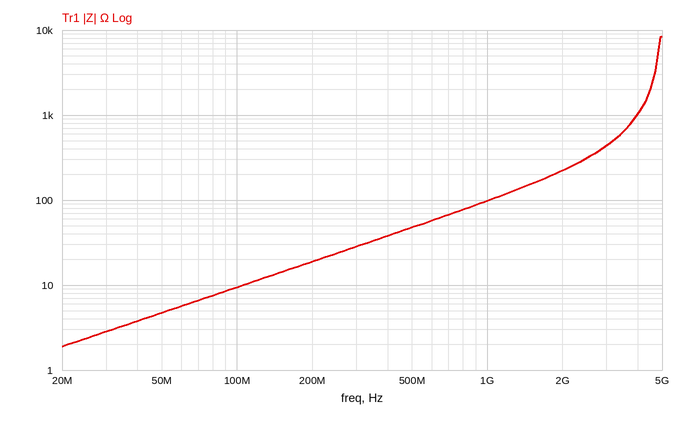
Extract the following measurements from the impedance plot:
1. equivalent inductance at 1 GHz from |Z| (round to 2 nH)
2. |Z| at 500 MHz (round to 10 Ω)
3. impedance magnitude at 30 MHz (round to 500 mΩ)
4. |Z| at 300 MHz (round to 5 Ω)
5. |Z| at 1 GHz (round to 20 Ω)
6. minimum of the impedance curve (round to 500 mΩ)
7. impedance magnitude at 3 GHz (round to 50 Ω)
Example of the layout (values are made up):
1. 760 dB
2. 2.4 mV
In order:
1. 16 nH
2. 50 Ω
3. 3.0 Ω
4. 30 Ω
5. 100 Ω
6. 2.0 Ω
7. 450 Ω
